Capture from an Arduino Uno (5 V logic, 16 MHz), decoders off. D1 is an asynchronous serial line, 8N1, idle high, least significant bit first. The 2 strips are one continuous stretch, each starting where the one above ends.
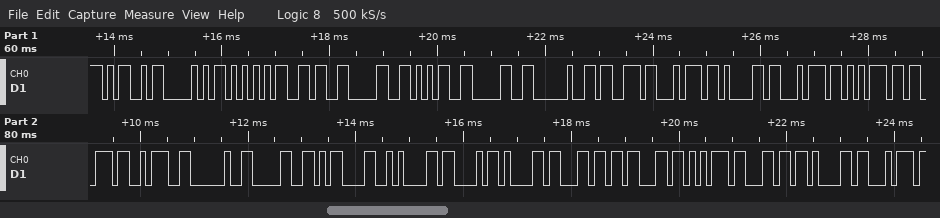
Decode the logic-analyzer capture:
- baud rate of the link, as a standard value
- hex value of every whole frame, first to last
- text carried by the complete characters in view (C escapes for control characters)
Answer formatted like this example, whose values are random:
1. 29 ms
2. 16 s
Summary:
1. 9600 baud
2. 0x4D 0x50 0x55 0x36 0x30 0x35 0x30 0x20 0x73 0x74 0x61 0x74 0x75 0x73 0x3A 0x20 0x30 0x0D 0x0A 0x43 0x61 0x6C 0x63 0x75 0x6C 0x61 0x74
3. "MPU6050 status: 0\r\nCalculat"
